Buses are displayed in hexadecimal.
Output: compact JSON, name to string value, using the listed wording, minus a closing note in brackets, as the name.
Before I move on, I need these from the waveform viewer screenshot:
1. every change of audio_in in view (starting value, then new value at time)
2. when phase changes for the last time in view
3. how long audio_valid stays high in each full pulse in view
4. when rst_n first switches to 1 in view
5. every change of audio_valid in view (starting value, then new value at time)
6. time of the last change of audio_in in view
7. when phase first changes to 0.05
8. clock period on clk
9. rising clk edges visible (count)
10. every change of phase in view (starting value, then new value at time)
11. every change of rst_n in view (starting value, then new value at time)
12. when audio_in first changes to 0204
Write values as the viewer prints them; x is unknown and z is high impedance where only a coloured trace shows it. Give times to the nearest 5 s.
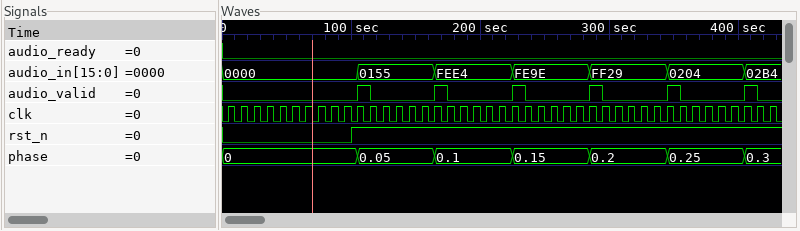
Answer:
{"every change of audio_in in view": "0000, 0155 at 105 s, FEE4 at 165 s, FE9E at 225 s, FF29 at 285 s, 0204 at 345 s, 02B4 at 405 s", "when phase changes for the last time in view": "405 s", "how long audio_valid stays high in each full pulse in view": "10 s, 10 s, 10 s, 10 s, 10 s, 10 s", "when rst_n first switches to 1 in view": "100 s", "every change of audio_valid in view": "0, 1 at 105 s, 0 at 115 s, 1 at 165 s, 0 at 175 s, 1 at 225 s, 0 at 235 s, 1 at 285 s, 0 at 295 s, 1 at 345 s, 0 at 355 s, 1 at 405 s, 0 at 415 s", "time of the last change of audio_in in view": "405 s", "when phase first changes to 0.05": "105 s", "clock period on clk": "10 s", "rising clk edges visible": "43", "every change of phase in view": "0, 0.05 at 105 s, 0.1 at 165 s, 0.15 at 225 s, 0.2 at 285 s, 0.25 at 345 s, 0.3 at 405 s", "every change of rst_n in view": "0, 1 at 100 s", "when audio_in first changes to 0204": "345 s"}
